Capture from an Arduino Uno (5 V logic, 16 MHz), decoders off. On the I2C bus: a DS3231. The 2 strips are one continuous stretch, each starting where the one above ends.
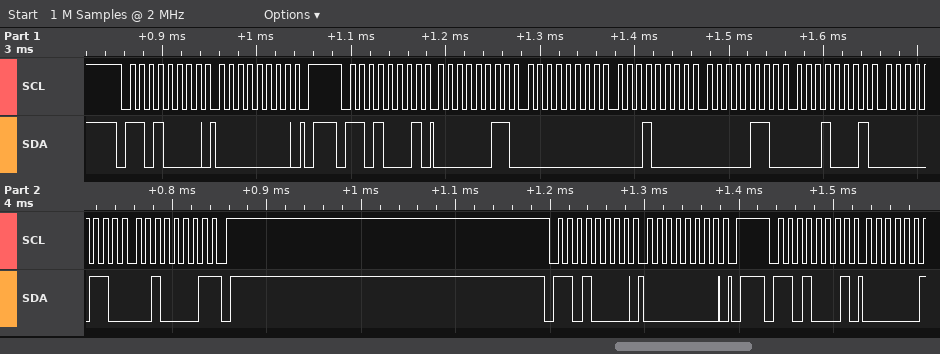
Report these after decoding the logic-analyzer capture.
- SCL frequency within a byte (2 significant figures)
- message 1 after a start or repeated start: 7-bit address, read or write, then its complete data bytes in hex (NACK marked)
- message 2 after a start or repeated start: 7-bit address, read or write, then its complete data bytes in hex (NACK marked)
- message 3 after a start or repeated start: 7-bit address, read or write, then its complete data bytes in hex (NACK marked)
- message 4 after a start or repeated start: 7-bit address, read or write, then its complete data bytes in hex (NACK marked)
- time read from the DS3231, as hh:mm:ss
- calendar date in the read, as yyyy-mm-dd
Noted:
100 kHz
0x68 write: 00
0x68 read: 03 00 10 06 11 06 21 NACK
0x68 write: 00
0x68 read
10:00:03
2021-06-11
